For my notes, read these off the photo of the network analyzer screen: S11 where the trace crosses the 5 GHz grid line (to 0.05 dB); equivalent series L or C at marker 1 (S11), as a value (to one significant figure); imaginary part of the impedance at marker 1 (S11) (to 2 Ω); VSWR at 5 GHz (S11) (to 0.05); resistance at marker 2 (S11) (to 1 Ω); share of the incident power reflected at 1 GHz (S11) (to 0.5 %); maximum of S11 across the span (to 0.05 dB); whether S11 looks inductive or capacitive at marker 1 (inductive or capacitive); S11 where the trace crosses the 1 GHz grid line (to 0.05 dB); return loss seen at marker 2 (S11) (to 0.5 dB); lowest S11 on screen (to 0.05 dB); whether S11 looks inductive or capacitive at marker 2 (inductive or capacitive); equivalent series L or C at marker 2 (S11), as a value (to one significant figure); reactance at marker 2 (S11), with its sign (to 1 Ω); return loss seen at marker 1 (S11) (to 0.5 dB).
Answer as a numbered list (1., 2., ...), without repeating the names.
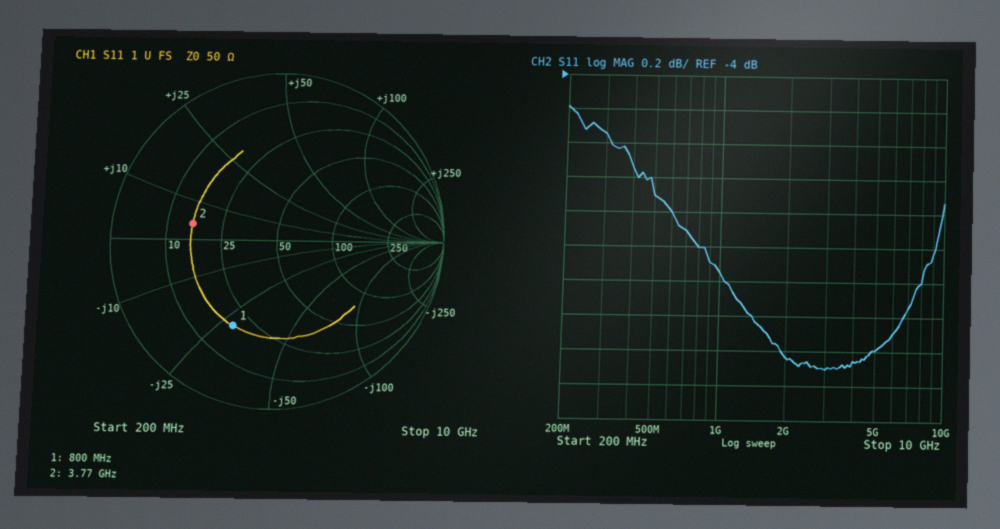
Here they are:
1. -5.60 dB
2. 7 pF
3. -28 Ω
4. 3.20
5. 16 Ω
6. 30.5 %
7. -4.20 dB
8. capacitive
9. -5.15 dB
10. 5.5 dB
11. -5.70 dB
12. inductive
13. 200 pH
14. +4 Ω
15. 5.0 dB
